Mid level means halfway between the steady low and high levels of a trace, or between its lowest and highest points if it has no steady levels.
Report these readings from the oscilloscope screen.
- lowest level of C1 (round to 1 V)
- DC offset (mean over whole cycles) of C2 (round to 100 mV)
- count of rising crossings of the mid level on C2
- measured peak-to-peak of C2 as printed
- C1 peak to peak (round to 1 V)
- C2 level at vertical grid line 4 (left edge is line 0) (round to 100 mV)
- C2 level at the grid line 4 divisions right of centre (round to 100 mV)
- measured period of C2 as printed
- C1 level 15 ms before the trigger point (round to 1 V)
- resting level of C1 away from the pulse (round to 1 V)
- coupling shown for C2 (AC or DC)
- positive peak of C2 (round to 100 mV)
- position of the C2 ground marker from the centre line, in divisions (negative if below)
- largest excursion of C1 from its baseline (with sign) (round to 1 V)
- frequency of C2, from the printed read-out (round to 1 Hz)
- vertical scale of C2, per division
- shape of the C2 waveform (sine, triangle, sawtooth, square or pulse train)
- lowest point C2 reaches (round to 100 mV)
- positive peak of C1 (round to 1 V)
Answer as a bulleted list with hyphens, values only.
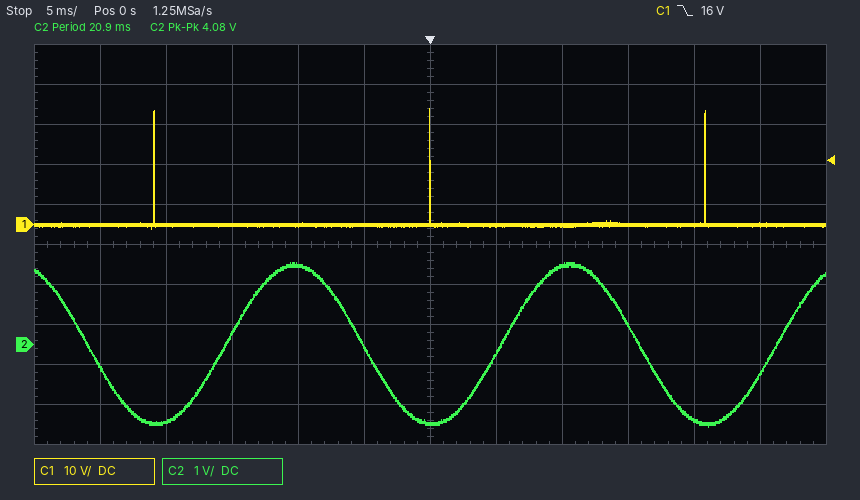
- -1 V
- 0.0 V
- 3
- 4.08 V
- 30 V
- 2.0 V
- -1.9 V
- 20.9 ms
- 0 V
- 0 V
- DC
- 2.0 V
- -2.5 div
- +29 V
- 48 Hz
- 1 V
- sine
- -2.0 V
- 29 V
